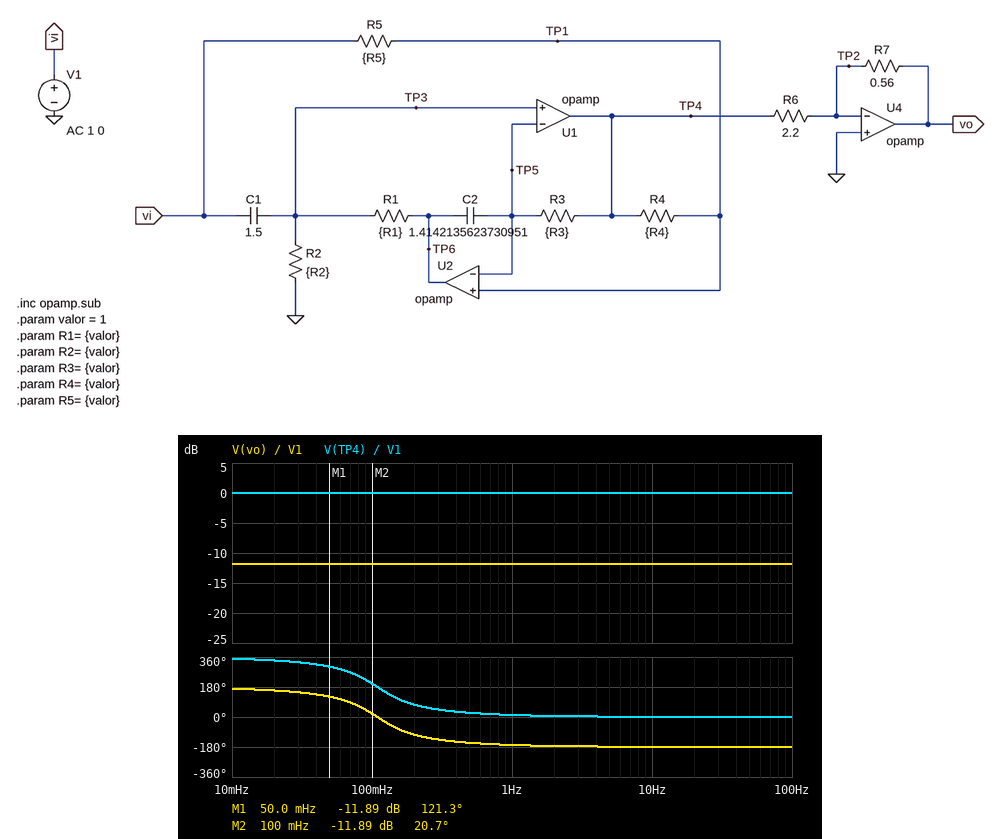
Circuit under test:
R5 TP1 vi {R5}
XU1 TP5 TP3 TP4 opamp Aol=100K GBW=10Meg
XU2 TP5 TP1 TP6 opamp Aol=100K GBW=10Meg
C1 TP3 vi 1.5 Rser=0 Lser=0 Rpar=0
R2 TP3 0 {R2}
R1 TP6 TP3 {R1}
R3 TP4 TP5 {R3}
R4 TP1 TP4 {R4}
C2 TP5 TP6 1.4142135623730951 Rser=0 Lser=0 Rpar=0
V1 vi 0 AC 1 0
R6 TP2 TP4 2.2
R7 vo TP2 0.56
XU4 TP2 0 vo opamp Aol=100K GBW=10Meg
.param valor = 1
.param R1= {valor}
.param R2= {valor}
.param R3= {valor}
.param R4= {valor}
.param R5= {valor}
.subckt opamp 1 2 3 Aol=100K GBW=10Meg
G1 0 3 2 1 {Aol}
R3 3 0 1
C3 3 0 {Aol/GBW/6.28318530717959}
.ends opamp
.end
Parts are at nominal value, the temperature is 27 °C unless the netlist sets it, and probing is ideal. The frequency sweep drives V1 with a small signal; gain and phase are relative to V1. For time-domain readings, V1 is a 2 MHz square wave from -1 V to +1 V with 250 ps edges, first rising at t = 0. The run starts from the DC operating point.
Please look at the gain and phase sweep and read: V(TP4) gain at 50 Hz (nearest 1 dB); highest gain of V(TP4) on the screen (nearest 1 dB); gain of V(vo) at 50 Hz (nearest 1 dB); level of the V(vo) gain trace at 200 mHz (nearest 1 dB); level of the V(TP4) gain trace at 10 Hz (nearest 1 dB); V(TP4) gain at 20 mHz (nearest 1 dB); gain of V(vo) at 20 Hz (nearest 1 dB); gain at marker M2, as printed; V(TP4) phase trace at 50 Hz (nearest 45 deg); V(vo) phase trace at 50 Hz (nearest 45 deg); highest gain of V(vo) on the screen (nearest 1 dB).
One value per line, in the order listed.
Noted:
0 dB
0 dB
-12 dB
-12 dB
0 dB
0 dB
-12 dB
-11.89 dB
0 deg
-180 deg
-12 dB
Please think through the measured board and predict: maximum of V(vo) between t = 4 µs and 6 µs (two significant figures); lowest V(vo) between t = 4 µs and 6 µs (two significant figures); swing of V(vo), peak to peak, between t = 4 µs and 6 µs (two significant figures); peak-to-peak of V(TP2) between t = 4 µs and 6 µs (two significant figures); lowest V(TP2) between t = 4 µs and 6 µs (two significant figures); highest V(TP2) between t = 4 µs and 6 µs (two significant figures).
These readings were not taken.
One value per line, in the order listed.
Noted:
310 mV
-310 mV
630 mV
420 mV
-210 mV
210 mV
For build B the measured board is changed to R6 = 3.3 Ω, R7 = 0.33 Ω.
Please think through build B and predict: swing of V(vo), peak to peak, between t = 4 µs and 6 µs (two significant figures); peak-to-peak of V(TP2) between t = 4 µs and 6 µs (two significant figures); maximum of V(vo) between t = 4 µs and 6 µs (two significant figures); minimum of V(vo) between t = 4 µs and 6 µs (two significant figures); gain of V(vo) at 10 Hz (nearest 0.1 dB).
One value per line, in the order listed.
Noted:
250 mV
180 mV
130 mV
-130 mV
-20.0 dB
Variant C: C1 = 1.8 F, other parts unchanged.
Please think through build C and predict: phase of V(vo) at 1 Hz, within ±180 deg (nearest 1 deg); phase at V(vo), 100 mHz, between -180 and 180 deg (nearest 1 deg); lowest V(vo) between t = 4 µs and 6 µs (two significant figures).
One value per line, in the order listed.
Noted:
-170 deg
-1 deg
-310 mV
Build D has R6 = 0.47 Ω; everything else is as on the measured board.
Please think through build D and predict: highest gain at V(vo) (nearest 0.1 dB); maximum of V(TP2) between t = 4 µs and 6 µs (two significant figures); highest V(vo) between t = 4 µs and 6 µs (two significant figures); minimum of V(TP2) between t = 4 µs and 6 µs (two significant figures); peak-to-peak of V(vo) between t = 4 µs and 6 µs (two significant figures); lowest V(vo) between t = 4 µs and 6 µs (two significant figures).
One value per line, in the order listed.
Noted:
1.5 dB
730 mV
1.3 V
-730 mV
2.5 V
-1.3 V
